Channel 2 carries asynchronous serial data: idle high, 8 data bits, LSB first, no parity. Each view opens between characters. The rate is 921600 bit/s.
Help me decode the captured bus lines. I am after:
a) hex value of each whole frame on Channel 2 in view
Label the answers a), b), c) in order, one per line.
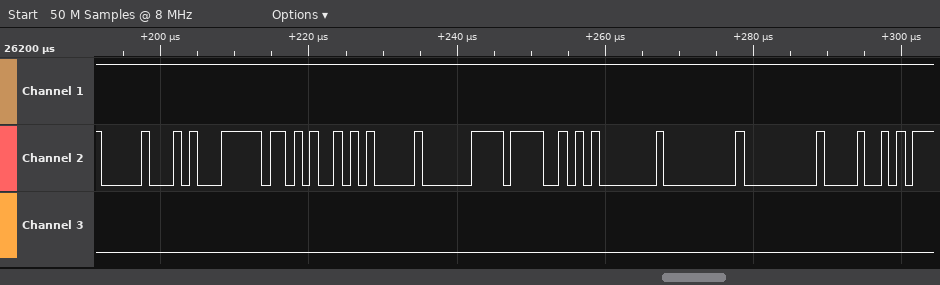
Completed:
a) 10, F1, 2B, 05, E0, 4F, 01, 00, 00, 48
